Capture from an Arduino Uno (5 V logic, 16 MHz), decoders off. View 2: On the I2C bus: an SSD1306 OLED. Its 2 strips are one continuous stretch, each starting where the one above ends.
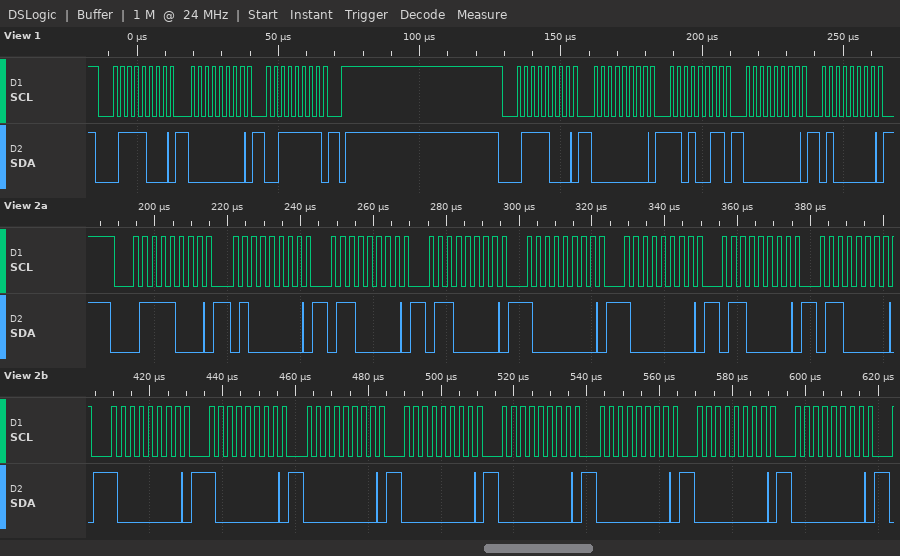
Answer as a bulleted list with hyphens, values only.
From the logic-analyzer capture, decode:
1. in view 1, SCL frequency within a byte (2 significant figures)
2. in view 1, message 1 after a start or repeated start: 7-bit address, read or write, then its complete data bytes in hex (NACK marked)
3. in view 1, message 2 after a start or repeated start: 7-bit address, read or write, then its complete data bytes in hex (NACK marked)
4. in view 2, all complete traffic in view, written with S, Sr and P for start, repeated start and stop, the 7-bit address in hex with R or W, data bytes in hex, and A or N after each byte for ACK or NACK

- 400 kHz
- 0x3C write: 00 3F
- 0x3C write: 00 D3 00 40
- S 3CW A 40 A 60 A 60 A 80 A 80 A 60 A 60 A 80 A 80 A 00 A 00 A 00 A 00 A 00 A 00 A
